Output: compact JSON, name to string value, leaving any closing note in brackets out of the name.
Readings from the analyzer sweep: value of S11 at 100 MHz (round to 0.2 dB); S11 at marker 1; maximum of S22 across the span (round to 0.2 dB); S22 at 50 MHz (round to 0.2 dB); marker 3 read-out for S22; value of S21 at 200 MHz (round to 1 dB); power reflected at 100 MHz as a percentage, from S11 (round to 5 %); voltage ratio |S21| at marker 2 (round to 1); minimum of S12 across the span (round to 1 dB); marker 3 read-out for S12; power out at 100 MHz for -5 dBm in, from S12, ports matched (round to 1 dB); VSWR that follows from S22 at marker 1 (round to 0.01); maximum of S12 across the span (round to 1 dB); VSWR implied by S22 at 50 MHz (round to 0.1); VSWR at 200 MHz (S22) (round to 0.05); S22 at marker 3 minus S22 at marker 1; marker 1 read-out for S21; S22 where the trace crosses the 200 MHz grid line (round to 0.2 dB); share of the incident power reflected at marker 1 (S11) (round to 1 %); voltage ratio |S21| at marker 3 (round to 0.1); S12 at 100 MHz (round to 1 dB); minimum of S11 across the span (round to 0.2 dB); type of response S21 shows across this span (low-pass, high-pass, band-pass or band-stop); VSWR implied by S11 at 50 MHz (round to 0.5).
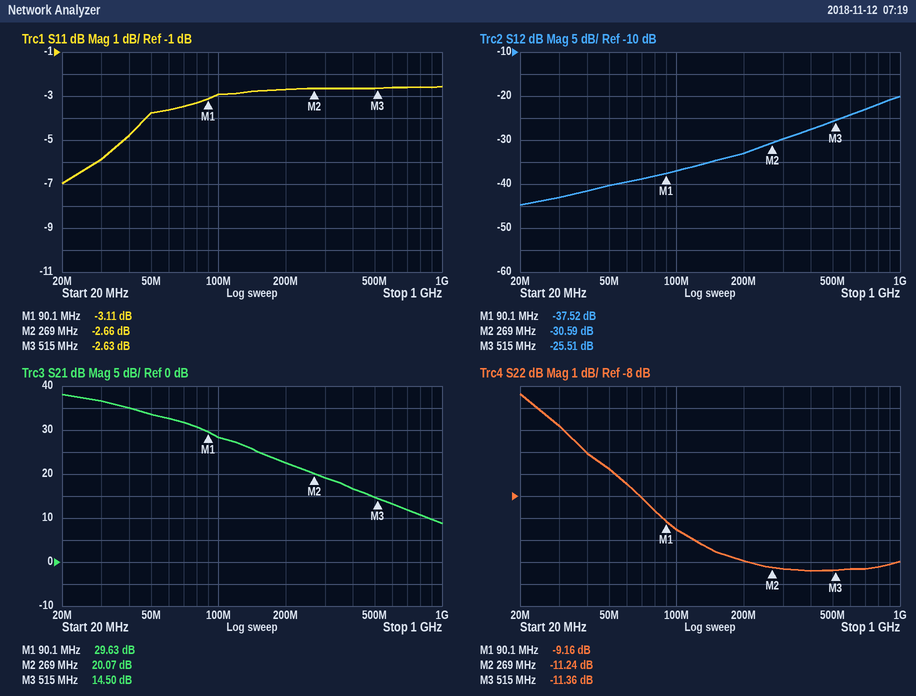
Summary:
{"value of S11 at 100 MHz": "-3.0 dB", "S11 at marker 1": "-3.11 dB", "maximum of S22 across the span": "-3.4 dB", "S22 at 50 MHz": "-6.8 dB", "marker 3 read-out for S22": "-11.36 dB", "value of S21 at 200 MHz": "23 dB", "power reflected at 100 MHz as a percentage, from S11": "50 %", "voltage ratio |S21| at marker 2": "10", "minimum of S12 across the span": "-45 dB", "marker 3 read-out for S12": "-25.51 dB", "power out at 100 MHz for -5 dBm in, from S12, ports matched": "-42 dBm", "VSWR that follows from S22 at marker 1": "2.07", "maximum of S12 across the span": "-20 dB", "VSWR implied by S22 at 50 MHz": "2.7", "VSWR at 200 MHz (S22)": "1.80", "S22 at marker 3 minus S22 at marker 1": "-2.20 dB", "marker 1 read-out for S21": "29.63 dB", "S22 where the trace crosses the 200 MHz grid line": "-11.0 dB", "share of the incident power reflected at marker 1 (S11)": "49 %", "voltage ratio |S21| at marker 3": "5.3", "S12 at 100 MHz": "-37 dB", "minimum of S11 across the span": "-7.0 dB", "type of response S21 shows across this span": "low-pass", "VSWR implied by S11 at 50 MHz": "4.5"}
